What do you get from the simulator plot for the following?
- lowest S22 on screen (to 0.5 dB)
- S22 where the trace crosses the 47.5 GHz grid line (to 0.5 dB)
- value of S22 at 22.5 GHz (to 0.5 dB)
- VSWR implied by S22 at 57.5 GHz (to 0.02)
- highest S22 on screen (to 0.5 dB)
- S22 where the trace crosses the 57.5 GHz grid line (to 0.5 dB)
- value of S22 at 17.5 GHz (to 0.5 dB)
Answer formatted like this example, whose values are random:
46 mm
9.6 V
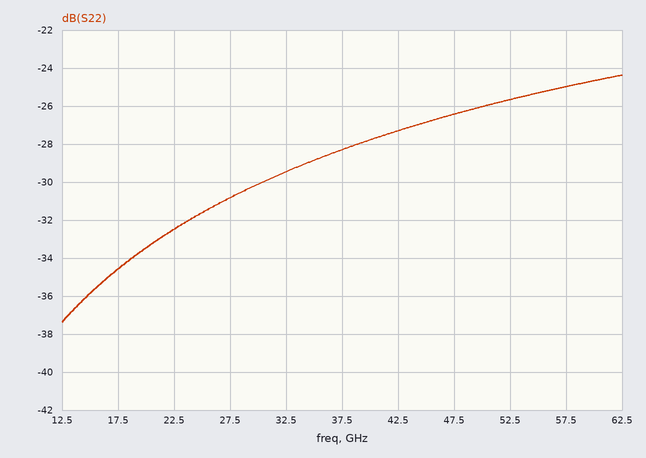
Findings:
-37.5 dB
-26.5 dB
-32.5 dB
1.12
-24.5 dB
-25.0 dB
-34.5 dB
